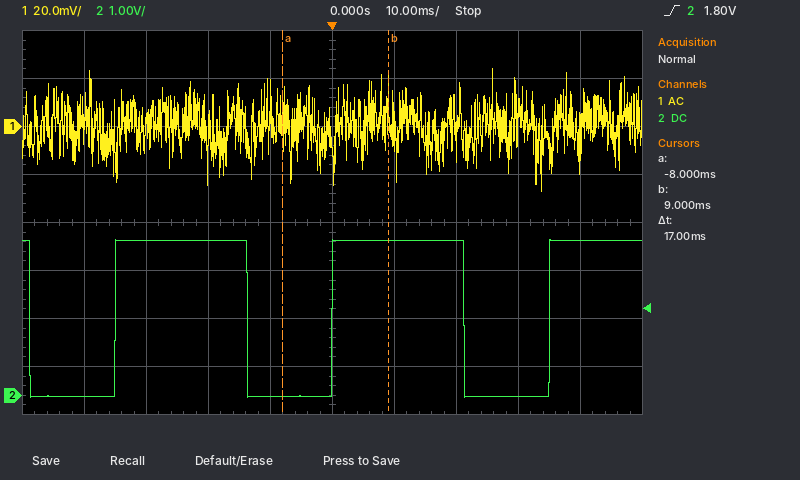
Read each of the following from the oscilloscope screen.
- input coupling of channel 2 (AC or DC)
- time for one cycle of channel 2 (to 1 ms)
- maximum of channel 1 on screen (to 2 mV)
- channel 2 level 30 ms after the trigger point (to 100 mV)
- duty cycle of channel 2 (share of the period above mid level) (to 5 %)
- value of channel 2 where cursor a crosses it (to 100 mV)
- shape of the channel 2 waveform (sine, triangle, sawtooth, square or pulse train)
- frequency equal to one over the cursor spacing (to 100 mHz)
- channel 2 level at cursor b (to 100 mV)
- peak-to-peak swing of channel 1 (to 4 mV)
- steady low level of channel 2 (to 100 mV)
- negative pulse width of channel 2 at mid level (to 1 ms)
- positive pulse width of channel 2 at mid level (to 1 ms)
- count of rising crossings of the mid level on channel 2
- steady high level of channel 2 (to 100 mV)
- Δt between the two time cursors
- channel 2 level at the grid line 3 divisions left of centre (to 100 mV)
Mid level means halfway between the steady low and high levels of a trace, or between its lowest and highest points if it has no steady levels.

DC
35 ms
24 mV
0.0 V
60 %
0.0 V
pulse train
58.8 Hz
3.2 V
52 mV
0.0 V
14 ms
21 ms
3
3.2 V
17 ms
3.2 V
